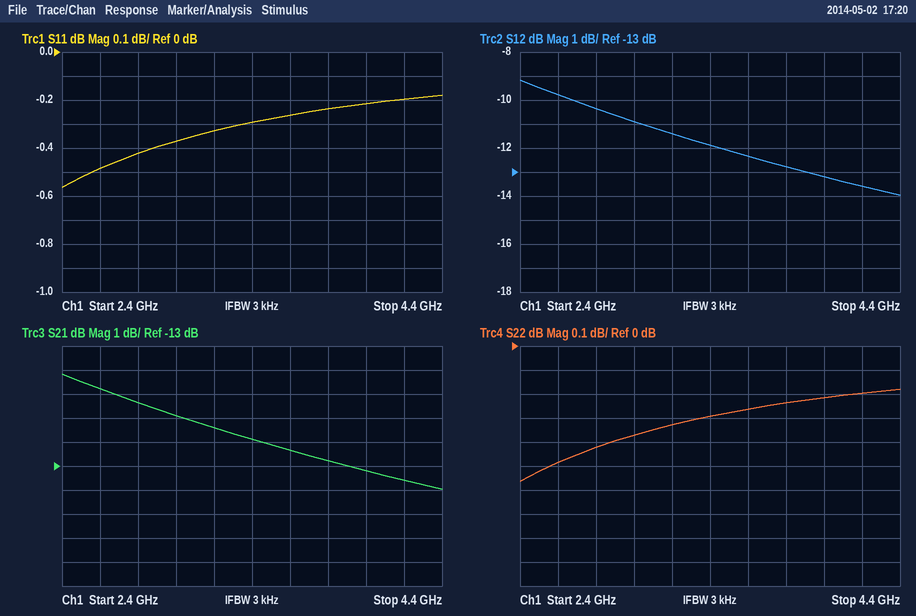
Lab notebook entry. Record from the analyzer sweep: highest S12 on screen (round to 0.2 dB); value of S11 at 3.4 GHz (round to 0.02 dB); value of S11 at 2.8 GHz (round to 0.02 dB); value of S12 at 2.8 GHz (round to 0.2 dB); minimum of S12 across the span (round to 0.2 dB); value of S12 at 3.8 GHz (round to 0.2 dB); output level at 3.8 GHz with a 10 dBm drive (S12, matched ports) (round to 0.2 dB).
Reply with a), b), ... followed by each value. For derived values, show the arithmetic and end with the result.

a) -9.2 dB
b) -0.30 dB
c) -0.42 dB
d) -10.4 dB
e) -14.0 dB
f) -12.8 dB
g) 10 dBm + (-12.8 dB) = -2.8 dBm
